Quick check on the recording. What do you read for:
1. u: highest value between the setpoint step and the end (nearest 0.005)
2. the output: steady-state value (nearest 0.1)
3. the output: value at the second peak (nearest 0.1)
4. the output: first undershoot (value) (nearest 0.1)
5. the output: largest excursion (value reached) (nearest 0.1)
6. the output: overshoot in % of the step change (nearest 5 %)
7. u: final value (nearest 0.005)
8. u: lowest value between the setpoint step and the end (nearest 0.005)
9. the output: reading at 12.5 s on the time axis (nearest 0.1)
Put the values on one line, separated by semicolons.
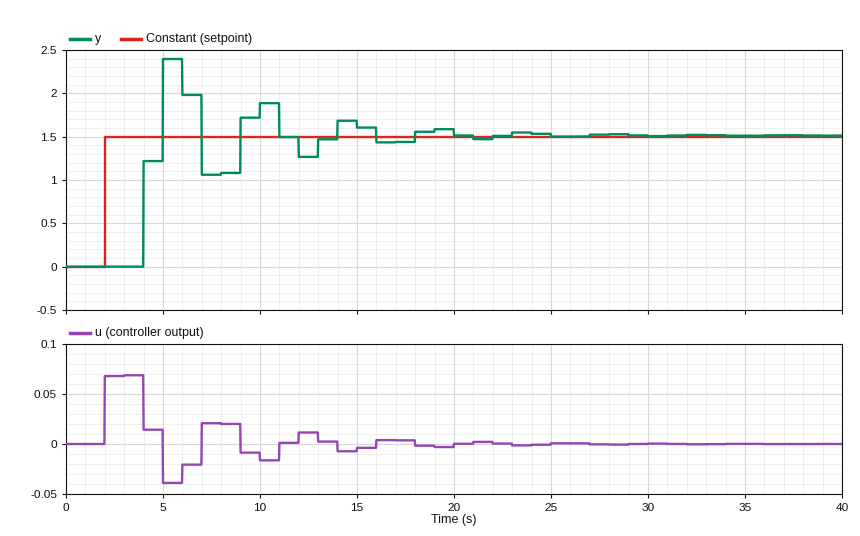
0.070; 1.5; 1.9; 1.1; 2.4; 60 %; 0.000; -0.040; 1.3
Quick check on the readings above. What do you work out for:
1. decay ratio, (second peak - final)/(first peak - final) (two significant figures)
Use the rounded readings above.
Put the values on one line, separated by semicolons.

0.44
